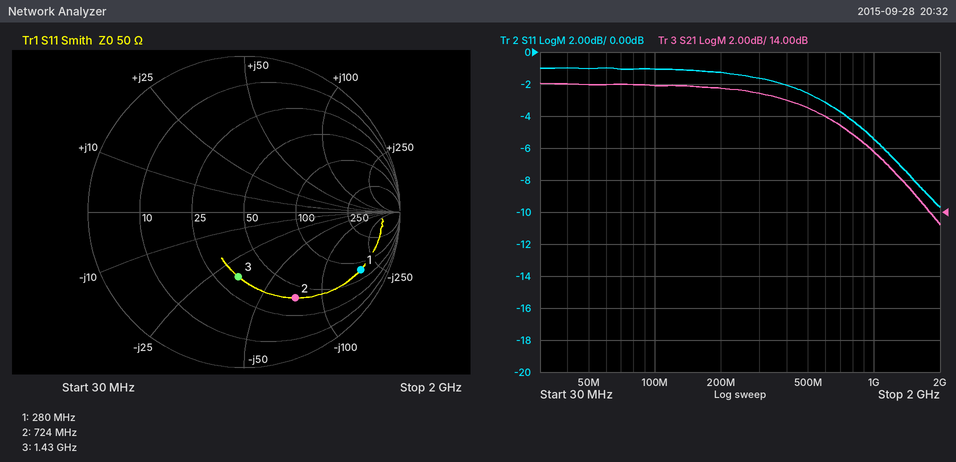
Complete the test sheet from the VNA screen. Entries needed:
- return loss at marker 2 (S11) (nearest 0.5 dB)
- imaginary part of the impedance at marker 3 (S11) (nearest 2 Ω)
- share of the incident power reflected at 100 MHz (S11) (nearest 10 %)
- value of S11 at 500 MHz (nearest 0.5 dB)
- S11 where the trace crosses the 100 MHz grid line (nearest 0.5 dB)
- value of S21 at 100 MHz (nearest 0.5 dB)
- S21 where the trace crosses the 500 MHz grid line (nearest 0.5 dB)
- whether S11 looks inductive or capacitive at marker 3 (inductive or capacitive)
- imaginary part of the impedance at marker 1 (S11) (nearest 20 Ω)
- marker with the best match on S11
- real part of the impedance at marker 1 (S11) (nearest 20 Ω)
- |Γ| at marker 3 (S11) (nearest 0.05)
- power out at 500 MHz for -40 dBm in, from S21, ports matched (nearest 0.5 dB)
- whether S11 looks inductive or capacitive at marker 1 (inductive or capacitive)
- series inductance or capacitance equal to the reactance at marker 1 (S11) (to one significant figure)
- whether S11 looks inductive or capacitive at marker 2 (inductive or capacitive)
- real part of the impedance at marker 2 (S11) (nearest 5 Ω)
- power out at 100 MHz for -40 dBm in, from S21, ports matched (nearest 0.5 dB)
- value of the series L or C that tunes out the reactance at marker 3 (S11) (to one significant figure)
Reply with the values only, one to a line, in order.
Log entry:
4.0 dB
-34 Ω
80 %
-2.5 dB
-1.0 dB
22.0 dB
20.5 dB
capacitive
-180 Ω
marker 3
80 Ω
0.40
-19.5 dBm
capacitive
3 pF
capacitive
40 Ω
-18.0 dBm
4 nH
